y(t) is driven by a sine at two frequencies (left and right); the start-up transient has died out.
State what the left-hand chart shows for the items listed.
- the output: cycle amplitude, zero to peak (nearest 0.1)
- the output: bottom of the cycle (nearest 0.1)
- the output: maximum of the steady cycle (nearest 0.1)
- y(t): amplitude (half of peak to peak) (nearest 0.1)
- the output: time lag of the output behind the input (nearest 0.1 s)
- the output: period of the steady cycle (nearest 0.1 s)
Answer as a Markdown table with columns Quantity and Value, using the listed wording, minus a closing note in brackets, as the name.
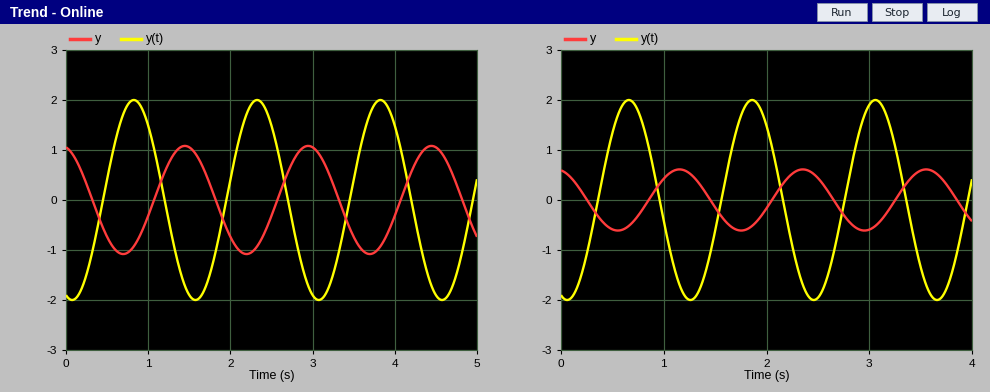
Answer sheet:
| Quantity | Value |
|---|---|
| the output: cycle amplitude, zero to peak | 1.1 |
| the output: bottom of the cycle | -1.1 |
| the output: maximum of the steady cycle | 1.1 |
| y(t): amplitude (half of peak to peak) | 2.0 |
| the output: time lag of the output behind the input | 0.6 s |
| the output: period of the steady cycle | 1.5 s |
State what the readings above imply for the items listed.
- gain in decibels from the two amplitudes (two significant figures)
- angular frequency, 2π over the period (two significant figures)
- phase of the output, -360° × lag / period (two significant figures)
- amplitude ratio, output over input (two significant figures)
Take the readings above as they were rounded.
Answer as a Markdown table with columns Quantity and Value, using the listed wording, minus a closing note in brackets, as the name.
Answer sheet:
| Quantity | Value |
|---|---|
| gain in decibels from the two amplitudes | -5.2 dB |
| angular frequency, 2π over the period | 4.2 rad/s |
| phase of the output, -360° × lag / period | -140° |
| amplitude ratio, output over input | 0.55 |
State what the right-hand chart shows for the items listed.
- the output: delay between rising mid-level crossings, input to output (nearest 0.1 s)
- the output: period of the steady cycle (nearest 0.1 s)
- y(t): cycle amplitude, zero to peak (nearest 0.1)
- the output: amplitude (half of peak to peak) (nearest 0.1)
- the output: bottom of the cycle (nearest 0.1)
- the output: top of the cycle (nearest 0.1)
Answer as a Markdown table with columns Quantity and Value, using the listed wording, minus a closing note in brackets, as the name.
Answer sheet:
| Quantity | Value |
|---|---|
| the output: delay between rising mid-level crossings, input to output | 0.5 s |
| the output: period of the steady cycle | 1.2 s |
| y(t): cycle amplitude, zero to peak | 2.0 |
| the output: amplitude (half of peak to peak) | 0.6 |
| the output: bottom of the cycle | -0.6 |
| the output: top of the cycle | 0.6 |
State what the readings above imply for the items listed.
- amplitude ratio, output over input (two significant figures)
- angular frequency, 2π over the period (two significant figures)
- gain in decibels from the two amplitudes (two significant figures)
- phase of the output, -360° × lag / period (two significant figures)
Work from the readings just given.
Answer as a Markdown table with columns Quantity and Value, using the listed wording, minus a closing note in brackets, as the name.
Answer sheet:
| Quantity | Value |
|---|---|
| amplitude ratio, output over input | 0.30 |
| angular frequency, 2π over the period | 5.2 rad/s |
| gain in decibels from the two amplitudes | -10 dB |
| phase of the output, -360° × lag / period | -150° |
